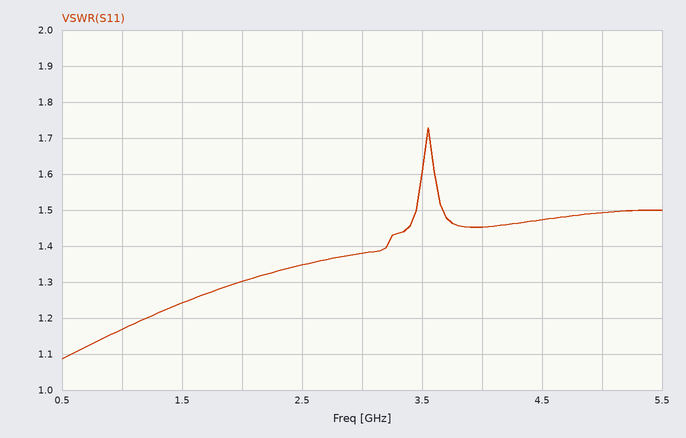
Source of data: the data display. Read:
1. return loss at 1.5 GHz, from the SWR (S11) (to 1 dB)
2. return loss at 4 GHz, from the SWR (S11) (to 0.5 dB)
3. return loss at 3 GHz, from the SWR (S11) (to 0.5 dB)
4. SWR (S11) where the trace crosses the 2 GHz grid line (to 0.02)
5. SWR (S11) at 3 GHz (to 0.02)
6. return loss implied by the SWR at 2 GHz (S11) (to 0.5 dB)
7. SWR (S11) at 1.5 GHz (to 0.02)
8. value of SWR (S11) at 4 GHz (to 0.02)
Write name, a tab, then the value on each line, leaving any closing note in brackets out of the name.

return loss at 1.5 GHz, from the SWR (S11)	19 dB
return loss at 4 GHz, from the SWR (S11)	14.5 dB
return loss at 3 GHz, from the SWR (S11)	16.0 dB
SWR (S11) where the trace crosses the 2 GHz grid line	1.30
SWR (S11) at 3 GHz	1.38
return loss implied by the SWR at 2 GHz (S11)	17.5 dB
SWR (S11) at 1.5 GHz	1.24
value of SWR (S11) at 4 GHz	1.46
